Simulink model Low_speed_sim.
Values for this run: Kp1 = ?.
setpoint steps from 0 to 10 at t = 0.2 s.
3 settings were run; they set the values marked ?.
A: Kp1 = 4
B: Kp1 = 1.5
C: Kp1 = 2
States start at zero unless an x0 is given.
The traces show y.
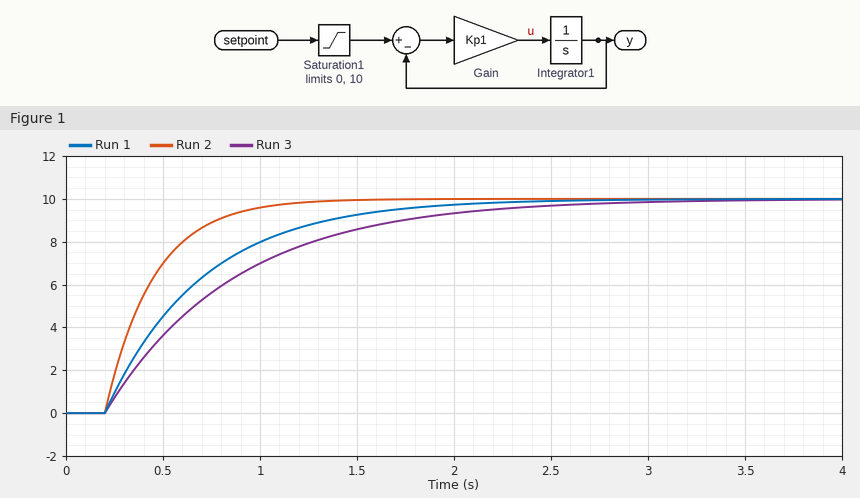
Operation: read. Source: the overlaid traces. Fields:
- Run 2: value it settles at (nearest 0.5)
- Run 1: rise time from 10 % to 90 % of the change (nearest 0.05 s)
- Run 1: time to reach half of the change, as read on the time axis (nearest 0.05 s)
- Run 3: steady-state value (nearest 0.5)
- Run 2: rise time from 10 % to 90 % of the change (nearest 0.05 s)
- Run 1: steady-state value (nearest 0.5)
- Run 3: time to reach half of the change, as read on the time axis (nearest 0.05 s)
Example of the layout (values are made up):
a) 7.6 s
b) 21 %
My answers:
a) 10.0
b) 1.10 s
c) 0.55 s
d) 10.0
e) 0.55 s
f) 10.0
g) 0.65 s
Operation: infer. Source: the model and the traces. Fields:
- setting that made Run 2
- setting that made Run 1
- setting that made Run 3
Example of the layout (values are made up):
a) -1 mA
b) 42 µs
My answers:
a) A
b) C
c) B
